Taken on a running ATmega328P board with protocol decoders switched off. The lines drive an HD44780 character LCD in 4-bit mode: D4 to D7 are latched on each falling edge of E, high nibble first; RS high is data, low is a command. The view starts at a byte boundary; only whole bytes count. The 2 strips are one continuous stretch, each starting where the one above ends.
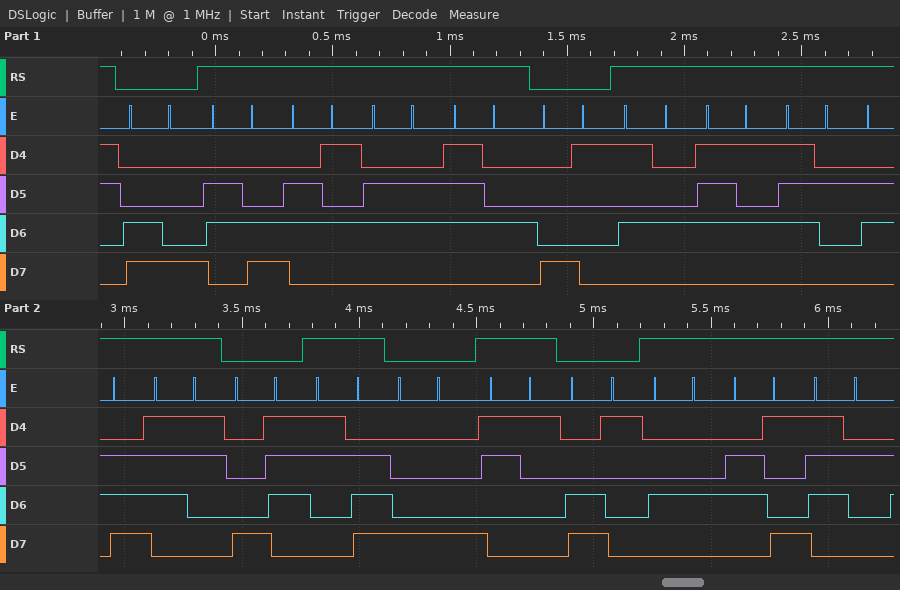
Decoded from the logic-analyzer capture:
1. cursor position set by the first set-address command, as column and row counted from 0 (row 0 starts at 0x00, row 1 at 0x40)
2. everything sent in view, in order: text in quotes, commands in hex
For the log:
column 8, row 1
0xC8 "left" 0x81 "Turns" 0x87 ">" 0x88 "1" 0xC1 "Dir"
